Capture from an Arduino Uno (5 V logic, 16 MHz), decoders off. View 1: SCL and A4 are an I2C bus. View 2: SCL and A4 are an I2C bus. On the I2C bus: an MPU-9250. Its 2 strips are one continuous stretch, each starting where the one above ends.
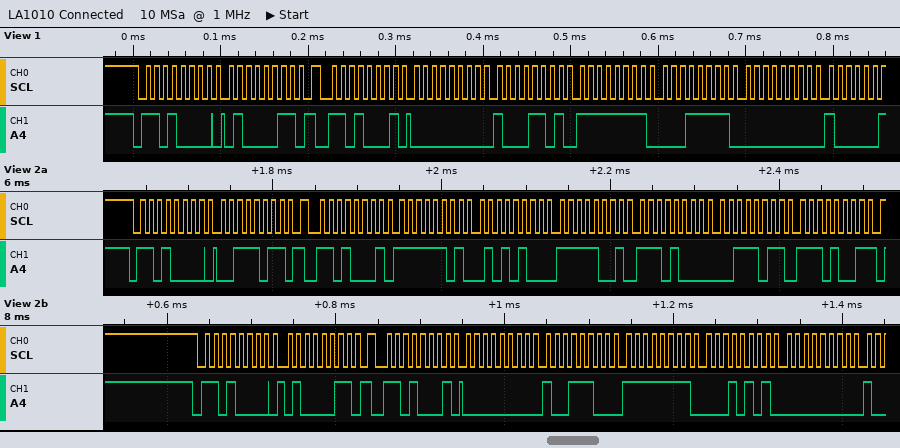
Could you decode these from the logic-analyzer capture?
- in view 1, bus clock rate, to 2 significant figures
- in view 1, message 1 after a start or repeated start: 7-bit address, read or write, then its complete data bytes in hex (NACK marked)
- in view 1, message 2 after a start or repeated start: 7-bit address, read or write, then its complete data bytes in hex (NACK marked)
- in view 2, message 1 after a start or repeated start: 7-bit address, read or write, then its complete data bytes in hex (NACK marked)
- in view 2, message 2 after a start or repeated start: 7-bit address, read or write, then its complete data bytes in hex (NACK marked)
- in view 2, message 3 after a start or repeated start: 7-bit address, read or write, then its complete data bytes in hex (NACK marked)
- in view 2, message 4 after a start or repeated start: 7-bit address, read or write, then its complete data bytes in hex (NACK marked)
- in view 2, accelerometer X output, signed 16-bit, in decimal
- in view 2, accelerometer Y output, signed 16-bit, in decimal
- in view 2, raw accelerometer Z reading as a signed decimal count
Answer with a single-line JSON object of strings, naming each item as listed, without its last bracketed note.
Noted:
{"in view 1, bus clock rate, to 2 significant figures": "100 kHz", "in view 1, message 1 after a start or repeated start: 7-bit address, read or write, then its complete data bytes in hex": "0x68 write: 43", "in view 1, message 2 after a start or repeated start: 7-bit address, read or write, then its complete data bytes in hex": "0x68 read: 00 8D FF 1F 00", "in view 2, message 1 after a start or repeated start: 7-bit address, read or write, then its complete data bytes in hex": "0x68 write: 3B", "in view 2, message 2 after a start or repeated start: 7-bit address, read or write, then its complete data bytes in hex": "0x68 read: FD 54 F9 E8 3B E9 NACK", "in view 2, message 3 after a start or repeated start: 7-bit address, read or write, then its complete data bytes in hex": "0x68 write: 43", "in view 2, message 4 after a start or repeated start: 7-bit address, read or write, then its complete data bytes in hex": "0x68 read: 00 9C FF 15 00", "in view 2, accelerometer X output, signed 16-bit, in decimal": "-684", "in view 2, accelerometer Y output, signed 16-bit, in decimal": "-1560", "in view 2, raw accelerometer Z reading as a signed decimal count": "15337"}
